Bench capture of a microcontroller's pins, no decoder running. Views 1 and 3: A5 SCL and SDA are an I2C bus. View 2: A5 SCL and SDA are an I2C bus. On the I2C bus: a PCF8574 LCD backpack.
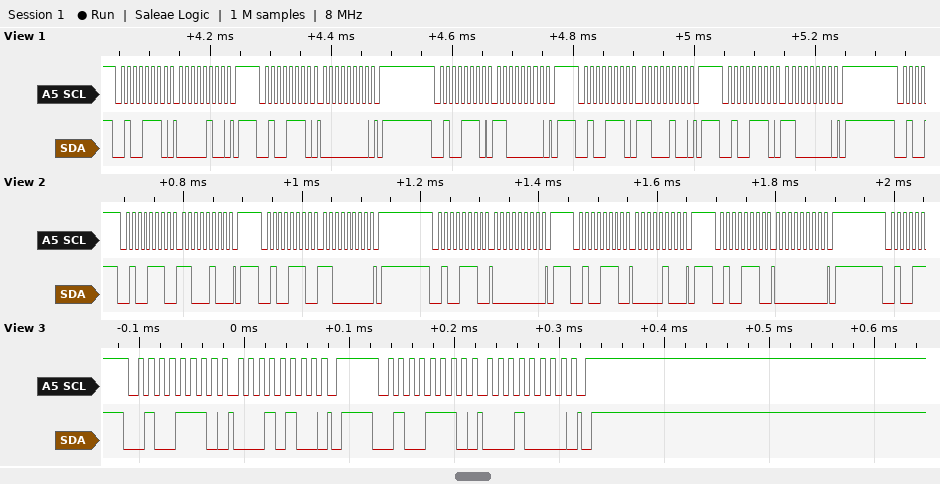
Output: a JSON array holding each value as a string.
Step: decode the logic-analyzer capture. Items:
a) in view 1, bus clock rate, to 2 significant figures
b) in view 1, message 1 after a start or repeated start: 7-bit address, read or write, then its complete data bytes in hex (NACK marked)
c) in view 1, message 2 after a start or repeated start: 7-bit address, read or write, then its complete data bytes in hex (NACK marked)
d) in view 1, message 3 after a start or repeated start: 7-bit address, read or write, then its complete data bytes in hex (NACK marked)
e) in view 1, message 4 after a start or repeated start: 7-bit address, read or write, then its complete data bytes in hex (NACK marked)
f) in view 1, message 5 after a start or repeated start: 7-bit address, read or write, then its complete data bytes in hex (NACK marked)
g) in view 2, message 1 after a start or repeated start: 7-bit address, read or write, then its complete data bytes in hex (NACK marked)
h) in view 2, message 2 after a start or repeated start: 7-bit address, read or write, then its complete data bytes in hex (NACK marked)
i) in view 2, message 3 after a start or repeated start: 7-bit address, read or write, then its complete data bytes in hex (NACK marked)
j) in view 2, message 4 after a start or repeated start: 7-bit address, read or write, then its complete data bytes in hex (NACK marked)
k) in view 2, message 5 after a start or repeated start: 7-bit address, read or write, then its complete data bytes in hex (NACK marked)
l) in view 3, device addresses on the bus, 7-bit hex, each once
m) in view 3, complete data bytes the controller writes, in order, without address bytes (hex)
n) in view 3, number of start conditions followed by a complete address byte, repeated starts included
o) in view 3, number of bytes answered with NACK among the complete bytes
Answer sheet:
["100 kHz", "0x27 write: 04", "0x27 write: 00", "0x27 write: C0", "0x27 write: C4", "0x27 write: C0", "0x27 write: C4", "0x27 write: C0", "0x27 write: 00", "0x27 write: 04", "0x27 write: 00", "0x27", "14 10", "2", "0"]
